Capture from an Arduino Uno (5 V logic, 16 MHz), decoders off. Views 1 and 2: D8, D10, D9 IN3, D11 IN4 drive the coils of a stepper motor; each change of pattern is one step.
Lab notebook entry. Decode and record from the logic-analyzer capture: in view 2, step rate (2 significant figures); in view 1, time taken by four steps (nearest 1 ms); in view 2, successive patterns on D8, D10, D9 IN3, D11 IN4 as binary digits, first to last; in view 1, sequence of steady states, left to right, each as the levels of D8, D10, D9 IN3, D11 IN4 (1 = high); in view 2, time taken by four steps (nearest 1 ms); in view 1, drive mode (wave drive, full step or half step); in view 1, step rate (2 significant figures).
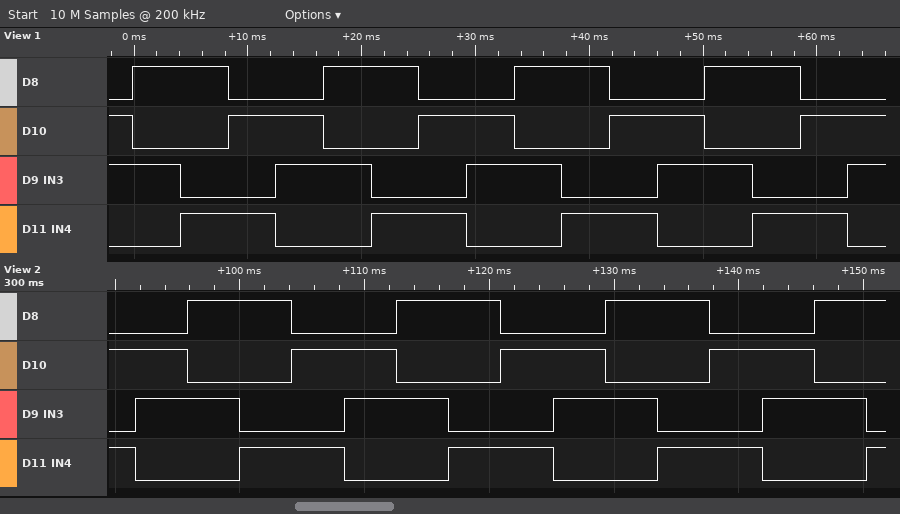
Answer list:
240 steps/s
17 ms
0101 0110 1010 1001 0101 0110 1010 1001 0101 0110 1010 1001 0101 0110 1010 1001
0110 1010 1001 0101 0110 1010 1001 0101 0110 1010 1001 0101 0110 1010 1001 0101 0110
17 ms
full step
240 steps/s
